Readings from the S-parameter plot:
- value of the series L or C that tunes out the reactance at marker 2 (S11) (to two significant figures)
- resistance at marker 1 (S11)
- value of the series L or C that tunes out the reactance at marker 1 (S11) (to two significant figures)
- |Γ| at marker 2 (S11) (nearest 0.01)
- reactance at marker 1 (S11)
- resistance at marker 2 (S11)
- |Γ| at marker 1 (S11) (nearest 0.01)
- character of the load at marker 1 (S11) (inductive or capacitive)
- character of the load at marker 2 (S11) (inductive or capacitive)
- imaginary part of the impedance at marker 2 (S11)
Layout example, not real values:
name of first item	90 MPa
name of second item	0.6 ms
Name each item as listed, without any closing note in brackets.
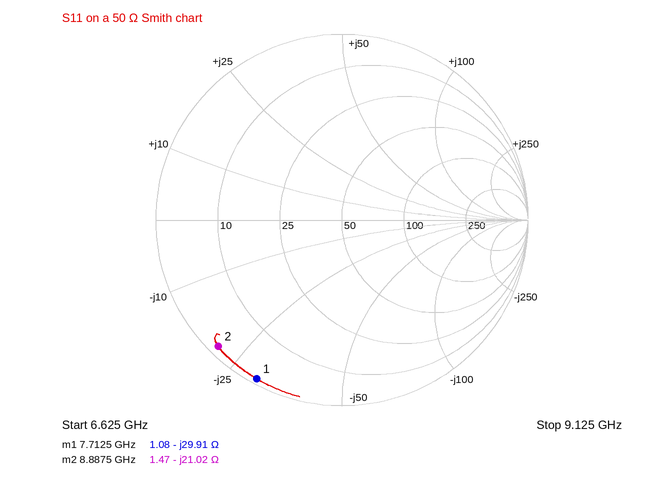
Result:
value of the series L or C that tunes out the reactance at marker 2 (S11)	380 pH
resistance at marker 1	1.08 Ω
value of the series L or C that tunes out the reactance at marker 1 (S11)	620 pH
|Γ| at marker 2 (S11)	0.95
reactance at marker 1	-29.91 Ω
resistance at marker 2	1.47 Ω
|Γ| at marker 1 (S11)	0.97
character of the load at marker 1 (S11)	capacitive
character of the load at marker 2 (S11)	capacitive
imaginary part of the impedance at marker 2	-21.02 Ω
